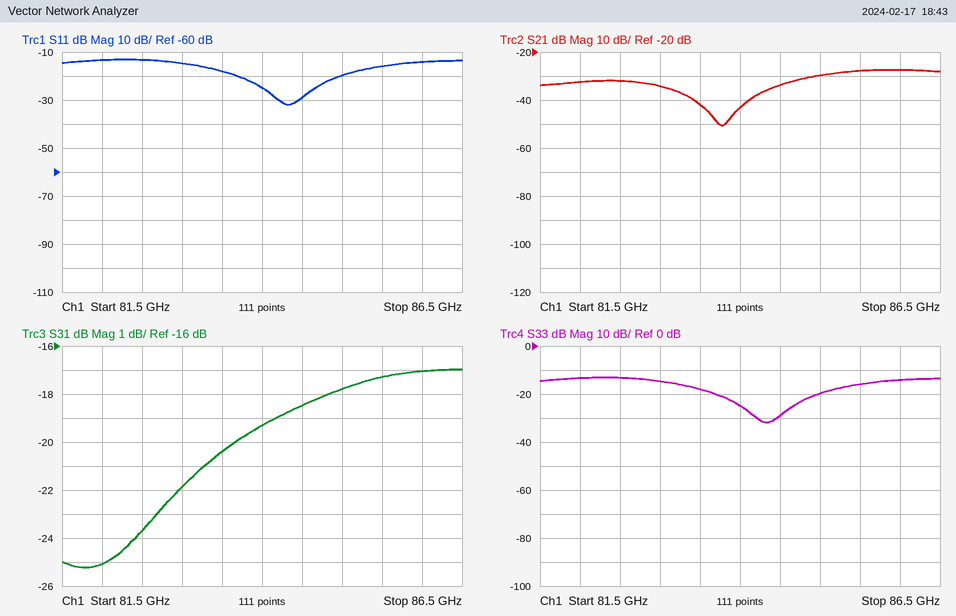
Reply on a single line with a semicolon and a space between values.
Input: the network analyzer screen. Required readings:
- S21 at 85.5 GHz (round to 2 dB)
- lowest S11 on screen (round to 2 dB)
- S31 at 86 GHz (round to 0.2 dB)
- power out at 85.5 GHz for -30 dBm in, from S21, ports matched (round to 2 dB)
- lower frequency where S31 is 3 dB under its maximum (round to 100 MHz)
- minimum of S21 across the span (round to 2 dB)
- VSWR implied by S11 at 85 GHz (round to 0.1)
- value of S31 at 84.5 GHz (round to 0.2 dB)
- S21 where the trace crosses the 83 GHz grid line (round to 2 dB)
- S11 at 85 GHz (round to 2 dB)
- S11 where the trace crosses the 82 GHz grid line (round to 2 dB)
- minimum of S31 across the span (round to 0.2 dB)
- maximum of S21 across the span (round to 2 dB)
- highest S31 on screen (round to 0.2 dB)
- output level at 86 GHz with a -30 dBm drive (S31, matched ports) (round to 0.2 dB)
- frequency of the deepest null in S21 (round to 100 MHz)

-28 dB; -32 dB; -17.0 dB; -58 dBm; 83.7 GHz; -50 dB; 1.2; -18.4 dB; -34 dB; -20 dB; -14 dB; -25.2 dB; -28 dB; -17.0 dB; -47.0 dBm; 83.8 GHz
